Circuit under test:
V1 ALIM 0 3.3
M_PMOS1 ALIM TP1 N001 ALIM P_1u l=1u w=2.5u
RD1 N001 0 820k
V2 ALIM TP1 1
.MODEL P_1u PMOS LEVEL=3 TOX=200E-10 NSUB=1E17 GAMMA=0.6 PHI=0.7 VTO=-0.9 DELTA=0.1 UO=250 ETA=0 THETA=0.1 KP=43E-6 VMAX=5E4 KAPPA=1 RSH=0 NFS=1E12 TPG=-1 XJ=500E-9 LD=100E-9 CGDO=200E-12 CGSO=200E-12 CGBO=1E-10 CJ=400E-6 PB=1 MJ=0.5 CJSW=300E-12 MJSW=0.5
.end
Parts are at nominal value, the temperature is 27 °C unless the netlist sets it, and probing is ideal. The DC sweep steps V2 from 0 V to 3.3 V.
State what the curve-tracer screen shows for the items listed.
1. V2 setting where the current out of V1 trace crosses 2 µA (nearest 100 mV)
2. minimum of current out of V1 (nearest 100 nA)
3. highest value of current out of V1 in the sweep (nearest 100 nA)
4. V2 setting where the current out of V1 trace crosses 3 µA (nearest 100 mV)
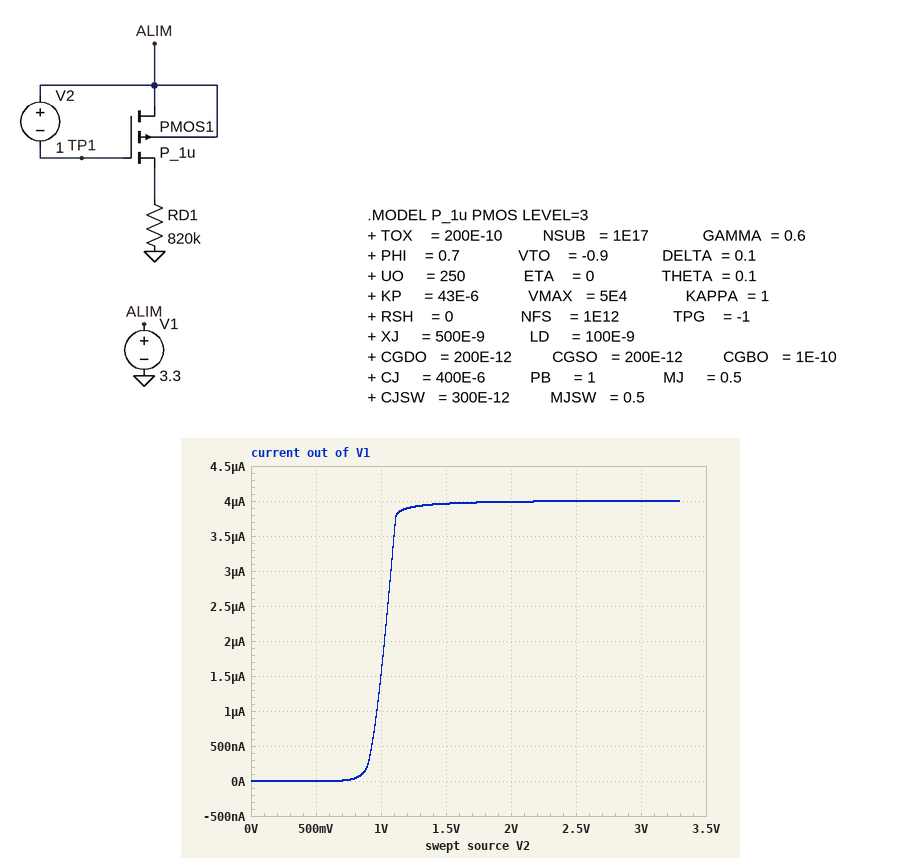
1.0 V
0 A
4.0 µA
1.1 V
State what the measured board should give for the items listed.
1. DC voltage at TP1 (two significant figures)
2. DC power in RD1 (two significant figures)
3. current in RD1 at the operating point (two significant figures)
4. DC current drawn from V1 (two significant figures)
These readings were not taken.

2.3 V
1.9 µW
1.5 µA
1.5 µA
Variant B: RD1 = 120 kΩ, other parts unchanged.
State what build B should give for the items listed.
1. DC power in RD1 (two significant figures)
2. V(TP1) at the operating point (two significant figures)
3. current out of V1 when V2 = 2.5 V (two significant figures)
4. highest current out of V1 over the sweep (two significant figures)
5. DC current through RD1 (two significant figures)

300 nW
2.3 V
26 µA
27 µA
1.6 µA
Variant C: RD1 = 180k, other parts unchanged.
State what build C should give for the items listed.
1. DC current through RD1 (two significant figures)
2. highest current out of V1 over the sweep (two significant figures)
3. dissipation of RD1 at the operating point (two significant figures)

1.6 µA
18 µA
440 nW
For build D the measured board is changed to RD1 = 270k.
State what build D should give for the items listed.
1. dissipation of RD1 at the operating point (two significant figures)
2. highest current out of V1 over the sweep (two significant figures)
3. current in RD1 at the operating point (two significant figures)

660 nW
12 µA
1.6 µA
